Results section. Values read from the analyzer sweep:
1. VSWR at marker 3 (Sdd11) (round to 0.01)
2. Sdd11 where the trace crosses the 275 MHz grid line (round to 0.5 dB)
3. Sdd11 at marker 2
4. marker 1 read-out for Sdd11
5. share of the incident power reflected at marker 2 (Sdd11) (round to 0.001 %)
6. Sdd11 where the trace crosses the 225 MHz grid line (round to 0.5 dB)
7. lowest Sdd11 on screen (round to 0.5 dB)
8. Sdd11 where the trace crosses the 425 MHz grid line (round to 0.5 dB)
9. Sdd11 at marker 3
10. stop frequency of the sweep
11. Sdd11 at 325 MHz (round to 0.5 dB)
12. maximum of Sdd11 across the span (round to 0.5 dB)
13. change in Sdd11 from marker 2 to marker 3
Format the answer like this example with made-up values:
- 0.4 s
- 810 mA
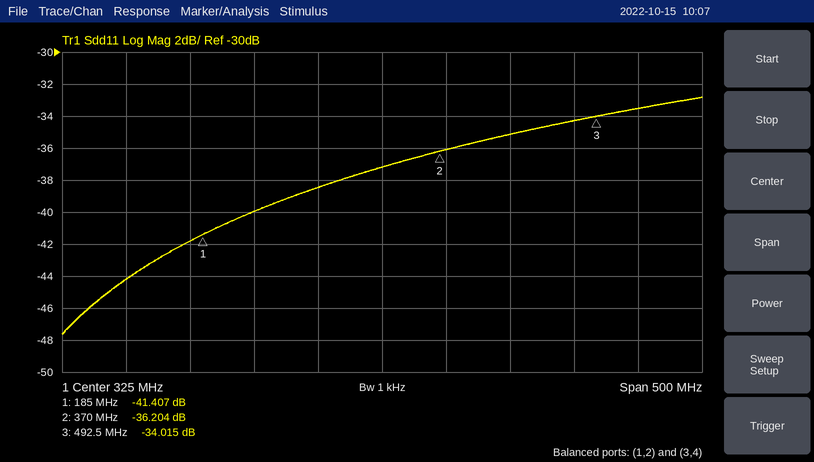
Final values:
- 1.04
- -38.5 dB
- -36.204 dB
- -41.407 dB
- 0.024 %
- -40.0 dB
- -47.5 dB
- -35.0 dB
- -34.015 dB
- 575 MHz
- -37.0 dB
- -33.0 dB
- 2.189 dB
